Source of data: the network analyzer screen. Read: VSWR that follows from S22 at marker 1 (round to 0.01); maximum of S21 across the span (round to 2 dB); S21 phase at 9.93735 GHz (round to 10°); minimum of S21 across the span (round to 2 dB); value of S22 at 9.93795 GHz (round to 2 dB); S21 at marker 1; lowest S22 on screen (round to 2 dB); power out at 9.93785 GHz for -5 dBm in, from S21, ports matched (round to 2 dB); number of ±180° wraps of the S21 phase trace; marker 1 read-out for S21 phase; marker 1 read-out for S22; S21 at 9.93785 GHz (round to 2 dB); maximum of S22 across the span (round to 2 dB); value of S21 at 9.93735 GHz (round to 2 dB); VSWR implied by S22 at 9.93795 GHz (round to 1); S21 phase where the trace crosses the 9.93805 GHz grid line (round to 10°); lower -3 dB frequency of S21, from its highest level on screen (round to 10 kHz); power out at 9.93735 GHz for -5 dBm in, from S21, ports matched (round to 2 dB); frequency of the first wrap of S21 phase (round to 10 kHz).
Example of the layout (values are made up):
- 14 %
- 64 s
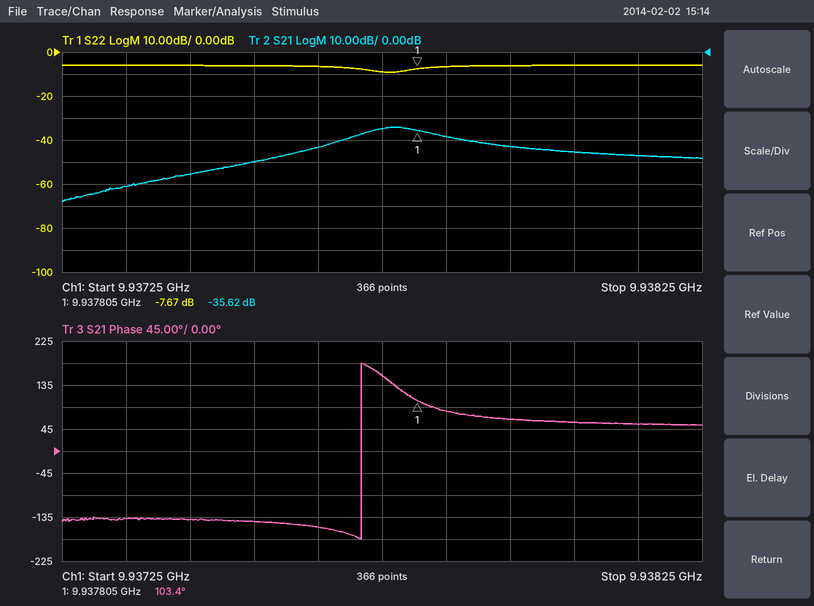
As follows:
- 2.41
- -34 dB
- -140°
- -68 dB
- -6 dB
- -35.62 dB
- -10 dB
- -44 dBm
- 1
- 103.4°
- -7.67 dB
- -38 dB
- -6 dB
- -62 dB
- 3
- 60°
- 9.93772 GHz
- -66 dBm
- 9.93772 GHz
